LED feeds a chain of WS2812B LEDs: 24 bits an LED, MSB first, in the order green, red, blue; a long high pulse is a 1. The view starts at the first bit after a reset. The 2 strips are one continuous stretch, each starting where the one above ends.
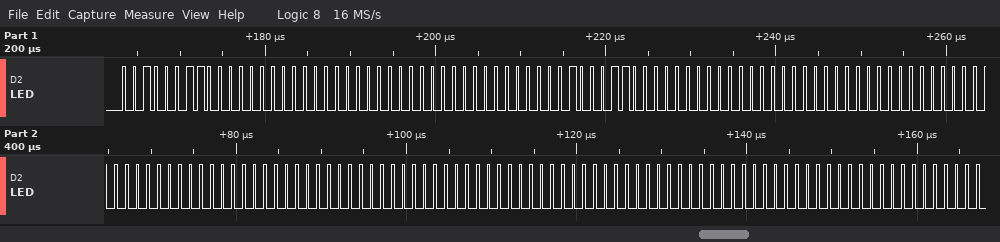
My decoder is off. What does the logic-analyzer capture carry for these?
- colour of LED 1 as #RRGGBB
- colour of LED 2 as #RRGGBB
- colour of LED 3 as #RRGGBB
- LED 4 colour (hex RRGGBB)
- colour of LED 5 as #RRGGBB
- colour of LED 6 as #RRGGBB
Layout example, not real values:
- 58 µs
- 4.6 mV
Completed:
- #002300
- #000023
- #000000
- #000000
- #000000
- #000000
